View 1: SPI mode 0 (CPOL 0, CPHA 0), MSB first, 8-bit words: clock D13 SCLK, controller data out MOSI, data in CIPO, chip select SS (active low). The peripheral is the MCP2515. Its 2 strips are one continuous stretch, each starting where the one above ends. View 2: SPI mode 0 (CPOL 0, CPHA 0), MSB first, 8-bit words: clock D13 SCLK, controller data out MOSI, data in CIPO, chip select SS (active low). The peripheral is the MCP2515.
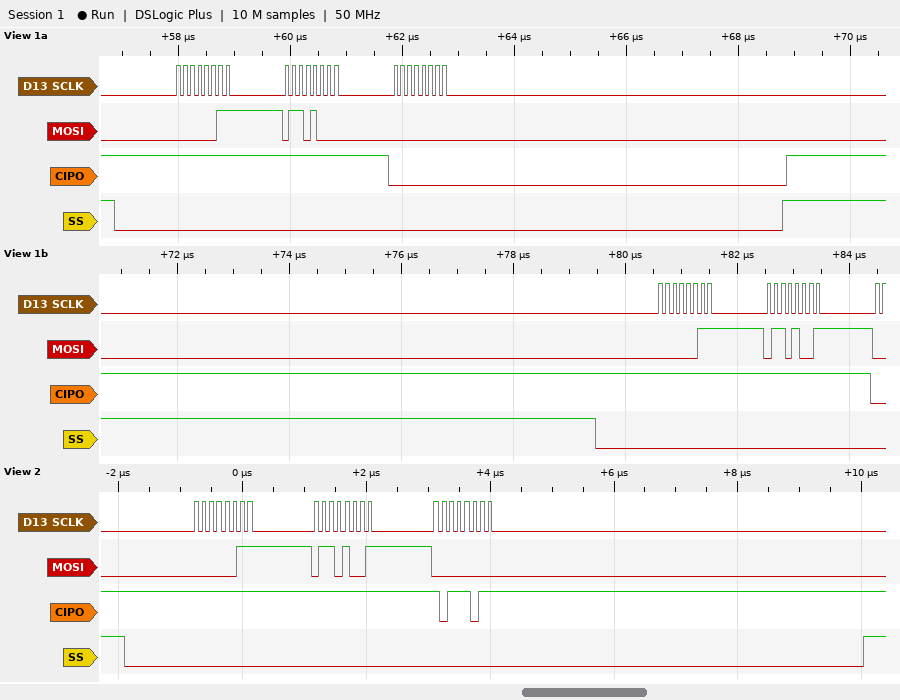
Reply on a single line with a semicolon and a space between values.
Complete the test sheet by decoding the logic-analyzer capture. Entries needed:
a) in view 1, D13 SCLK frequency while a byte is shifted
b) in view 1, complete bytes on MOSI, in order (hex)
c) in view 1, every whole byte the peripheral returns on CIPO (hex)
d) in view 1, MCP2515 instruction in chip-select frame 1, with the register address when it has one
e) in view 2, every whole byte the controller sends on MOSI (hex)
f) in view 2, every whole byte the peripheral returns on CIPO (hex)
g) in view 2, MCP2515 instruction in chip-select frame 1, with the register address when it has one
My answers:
8 MHz; 03 68 00 03 69; FF FF 00 FF FF; READ 0x68; 03 69 00; FF FF BB; READ 0x69
